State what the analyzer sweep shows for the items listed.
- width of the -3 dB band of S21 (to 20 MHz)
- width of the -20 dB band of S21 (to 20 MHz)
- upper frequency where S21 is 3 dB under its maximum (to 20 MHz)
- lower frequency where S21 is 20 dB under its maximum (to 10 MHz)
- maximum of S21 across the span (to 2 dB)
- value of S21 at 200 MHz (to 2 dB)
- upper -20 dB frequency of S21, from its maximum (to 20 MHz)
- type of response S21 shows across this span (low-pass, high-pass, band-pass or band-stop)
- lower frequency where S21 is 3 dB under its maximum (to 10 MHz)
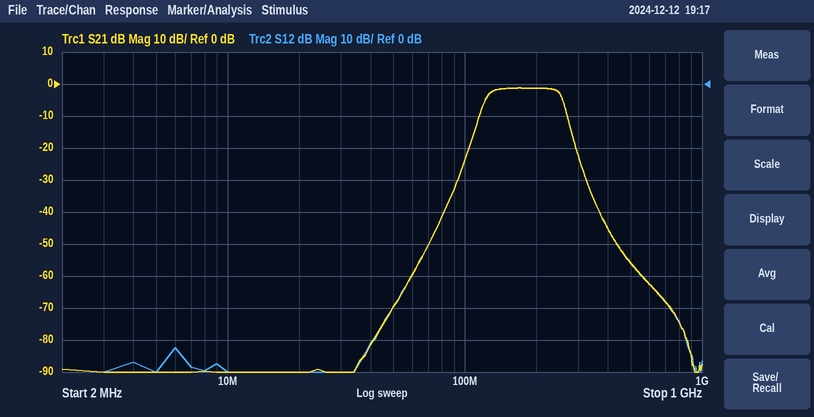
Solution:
140 MHz
200 MHz
260 MHz
100 MHz
-2 dB
-2 dB
300 MHz
band-pass
120 MHz
